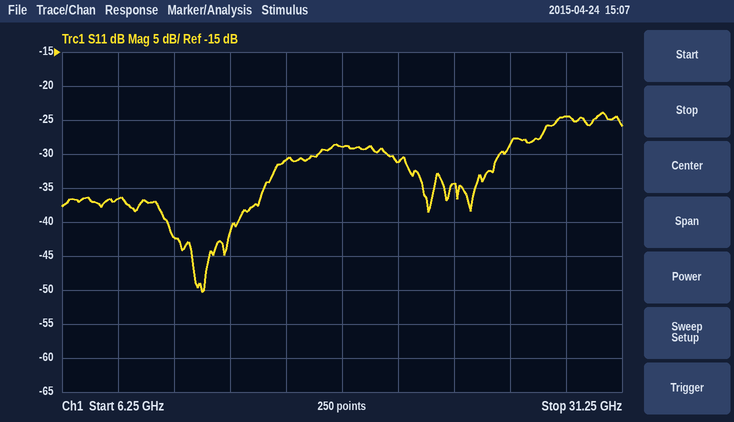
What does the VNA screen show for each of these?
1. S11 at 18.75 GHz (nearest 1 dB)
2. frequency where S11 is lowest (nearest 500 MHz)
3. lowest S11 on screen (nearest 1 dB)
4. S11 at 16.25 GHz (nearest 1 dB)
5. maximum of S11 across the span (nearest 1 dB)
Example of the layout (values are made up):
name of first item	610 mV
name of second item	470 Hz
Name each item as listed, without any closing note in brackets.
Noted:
S11 at 18.75 GHz	-29 dB
frequency where S11 is lowest	12.5 GHz
lowest S11 on screen	-50 dB
S11 at 16.25 GHz	-31 dB
maximum of S11 across the span	-24 dB
